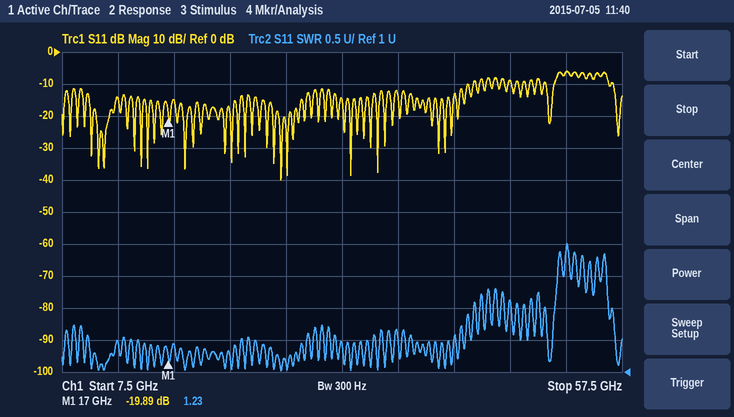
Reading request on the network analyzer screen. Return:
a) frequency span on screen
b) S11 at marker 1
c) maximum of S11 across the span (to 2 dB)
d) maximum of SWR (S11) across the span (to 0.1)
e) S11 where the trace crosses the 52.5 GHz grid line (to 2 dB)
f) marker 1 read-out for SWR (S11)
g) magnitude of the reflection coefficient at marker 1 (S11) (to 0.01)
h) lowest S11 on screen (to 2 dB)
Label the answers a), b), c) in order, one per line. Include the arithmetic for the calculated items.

a) 50 GHz
b) -19.89 dB
c) -6 dB
d) 3.0
e) -6 dB
f) 1.23
g) 10^(-19.89/20) ≈ 0.10
h) -40 dB
